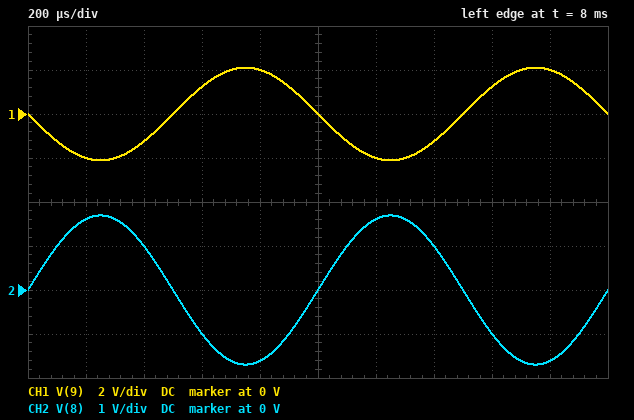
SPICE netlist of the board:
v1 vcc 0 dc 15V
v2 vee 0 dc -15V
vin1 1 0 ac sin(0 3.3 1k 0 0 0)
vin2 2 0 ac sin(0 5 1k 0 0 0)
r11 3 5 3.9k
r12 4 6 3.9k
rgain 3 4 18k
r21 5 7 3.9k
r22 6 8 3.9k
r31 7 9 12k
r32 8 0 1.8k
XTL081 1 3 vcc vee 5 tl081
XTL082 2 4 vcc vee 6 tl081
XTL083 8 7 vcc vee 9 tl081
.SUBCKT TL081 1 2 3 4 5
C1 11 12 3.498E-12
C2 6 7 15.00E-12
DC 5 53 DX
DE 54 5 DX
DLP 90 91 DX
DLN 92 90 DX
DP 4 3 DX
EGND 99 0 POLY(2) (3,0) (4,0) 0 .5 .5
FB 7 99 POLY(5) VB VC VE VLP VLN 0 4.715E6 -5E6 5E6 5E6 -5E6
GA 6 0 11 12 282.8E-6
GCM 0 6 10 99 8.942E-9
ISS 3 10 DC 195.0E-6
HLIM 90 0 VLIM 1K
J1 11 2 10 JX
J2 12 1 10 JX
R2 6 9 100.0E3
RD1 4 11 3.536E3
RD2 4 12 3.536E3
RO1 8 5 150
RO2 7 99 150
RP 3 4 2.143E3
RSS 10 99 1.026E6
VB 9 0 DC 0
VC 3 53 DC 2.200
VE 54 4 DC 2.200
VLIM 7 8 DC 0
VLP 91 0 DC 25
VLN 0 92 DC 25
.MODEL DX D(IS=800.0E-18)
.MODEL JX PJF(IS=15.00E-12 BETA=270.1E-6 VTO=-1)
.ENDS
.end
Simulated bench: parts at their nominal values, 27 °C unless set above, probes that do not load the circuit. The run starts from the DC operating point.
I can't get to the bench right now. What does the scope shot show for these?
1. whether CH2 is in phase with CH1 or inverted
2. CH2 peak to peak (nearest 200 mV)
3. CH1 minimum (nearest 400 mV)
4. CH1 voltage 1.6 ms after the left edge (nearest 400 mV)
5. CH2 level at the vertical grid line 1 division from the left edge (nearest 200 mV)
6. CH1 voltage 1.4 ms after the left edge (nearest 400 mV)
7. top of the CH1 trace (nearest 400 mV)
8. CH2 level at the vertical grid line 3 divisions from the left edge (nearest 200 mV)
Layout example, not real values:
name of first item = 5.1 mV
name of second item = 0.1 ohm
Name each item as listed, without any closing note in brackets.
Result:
whether CH2 is in phase with CH1 or inverted = inverted
CH2 peak to peak = 3.4 V
CH1 minimum = -2.0 V
CH1 voltage 1.6 ms after the left edge = 1.2 V
CH2 level at the vertical grid line 1 division from the left edge = 1.6 V
CH1 voltage 1.4 ms after the left edge = -1.2 V
top of the CH1 trace = 2.0 V
CH2 level at the vertical grid line 3 divisions from the left edge = -1.0 V
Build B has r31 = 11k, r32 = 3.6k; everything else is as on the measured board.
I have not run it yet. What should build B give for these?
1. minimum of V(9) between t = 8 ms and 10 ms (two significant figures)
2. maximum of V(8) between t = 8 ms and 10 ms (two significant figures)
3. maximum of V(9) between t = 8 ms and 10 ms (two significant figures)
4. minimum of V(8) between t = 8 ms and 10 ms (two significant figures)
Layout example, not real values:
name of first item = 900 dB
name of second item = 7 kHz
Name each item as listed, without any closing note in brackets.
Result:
minimum of V(9) between t = 8 ms and 10 ms = -1.6 V
maximum of V(8) between t = 8 ms and 10 ms = 2.6 V
maximum of V(9) between t = 8 ms and 10 ms = 1.6 V
minimum of V(8) between t = 8 ms and 10 ms = -2.6 V
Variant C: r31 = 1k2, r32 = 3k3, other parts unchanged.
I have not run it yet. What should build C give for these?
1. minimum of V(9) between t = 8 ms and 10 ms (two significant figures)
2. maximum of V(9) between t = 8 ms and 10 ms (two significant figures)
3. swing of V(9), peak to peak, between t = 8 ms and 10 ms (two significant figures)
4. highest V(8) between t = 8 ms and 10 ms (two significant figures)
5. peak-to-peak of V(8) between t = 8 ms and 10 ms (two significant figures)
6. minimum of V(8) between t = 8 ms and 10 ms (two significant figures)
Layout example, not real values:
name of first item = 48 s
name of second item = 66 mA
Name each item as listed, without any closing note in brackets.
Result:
minimum of V(9) between t = 8 ms and 10 ms = -2.3 V
maximum of V(9) between t = 8 ms and 10 ms = 2.3 V
swing of V(9), peak to peak, between t = 8 ms and 10 ms = 4.6 V
highest V(8) between t = 8 ms and 10 ms = 2.5 V
peak-to-peak of V(8) between t = 8 ms and 10 ms = 4.9 V
minimum of V(8) between t = 8 ms and 10 ms = -2.5 V
